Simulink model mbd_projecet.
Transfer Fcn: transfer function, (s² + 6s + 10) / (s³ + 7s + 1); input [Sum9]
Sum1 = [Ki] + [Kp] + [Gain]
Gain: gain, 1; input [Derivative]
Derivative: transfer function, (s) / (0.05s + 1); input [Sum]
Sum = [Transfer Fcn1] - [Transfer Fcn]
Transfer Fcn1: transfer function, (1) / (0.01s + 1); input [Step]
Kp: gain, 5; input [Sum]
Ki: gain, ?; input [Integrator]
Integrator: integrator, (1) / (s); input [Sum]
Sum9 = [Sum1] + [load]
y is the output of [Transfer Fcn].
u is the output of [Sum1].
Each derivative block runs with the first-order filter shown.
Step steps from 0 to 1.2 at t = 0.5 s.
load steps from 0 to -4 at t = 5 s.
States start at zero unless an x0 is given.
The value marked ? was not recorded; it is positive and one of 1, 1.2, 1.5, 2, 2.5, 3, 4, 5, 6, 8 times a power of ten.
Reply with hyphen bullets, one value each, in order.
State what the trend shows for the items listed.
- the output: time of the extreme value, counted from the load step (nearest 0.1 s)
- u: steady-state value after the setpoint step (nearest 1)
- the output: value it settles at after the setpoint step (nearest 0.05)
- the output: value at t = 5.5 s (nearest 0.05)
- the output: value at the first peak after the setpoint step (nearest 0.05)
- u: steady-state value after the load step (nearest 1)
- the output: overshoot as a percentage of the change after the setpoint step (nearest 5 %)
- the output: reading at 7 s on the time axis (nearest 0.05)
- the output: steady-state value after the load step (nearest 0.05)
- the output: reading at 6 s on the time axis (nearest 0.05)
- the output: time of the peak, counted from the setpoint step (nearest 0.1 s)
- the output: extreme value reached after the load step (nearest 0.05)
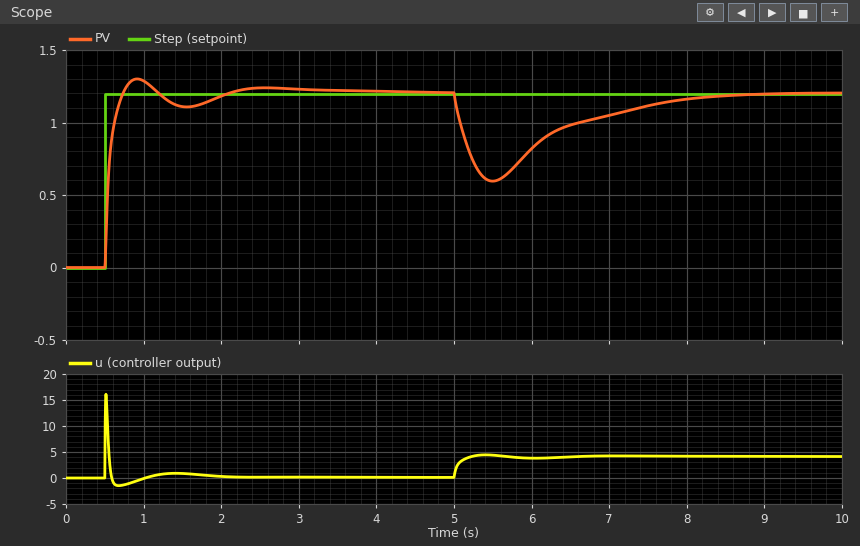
- 0.5 s
- 0
- 1.20
- 0.60
- 1.30
- 4
- 10 %
- 1.05
- 1.20
- 0.80
- 0.4 s
- 0.60
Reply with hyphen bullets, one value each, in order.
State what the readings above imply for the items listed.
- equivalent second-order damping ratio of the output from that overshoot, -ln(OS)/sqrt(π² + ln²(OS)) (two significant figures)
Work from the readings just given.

- 0.59
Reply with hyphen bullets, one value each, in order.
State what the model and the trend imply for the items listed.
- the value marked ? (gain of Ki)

- 5
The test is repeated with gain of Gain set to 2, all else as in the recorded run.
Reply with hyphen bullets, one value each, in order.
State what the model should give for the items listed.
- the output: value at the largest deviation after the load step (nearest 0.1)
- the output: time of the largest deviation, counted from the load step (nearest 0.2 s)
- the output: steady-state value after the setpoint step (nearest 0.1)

- 0.7
- 0.6 s
- 1.2
